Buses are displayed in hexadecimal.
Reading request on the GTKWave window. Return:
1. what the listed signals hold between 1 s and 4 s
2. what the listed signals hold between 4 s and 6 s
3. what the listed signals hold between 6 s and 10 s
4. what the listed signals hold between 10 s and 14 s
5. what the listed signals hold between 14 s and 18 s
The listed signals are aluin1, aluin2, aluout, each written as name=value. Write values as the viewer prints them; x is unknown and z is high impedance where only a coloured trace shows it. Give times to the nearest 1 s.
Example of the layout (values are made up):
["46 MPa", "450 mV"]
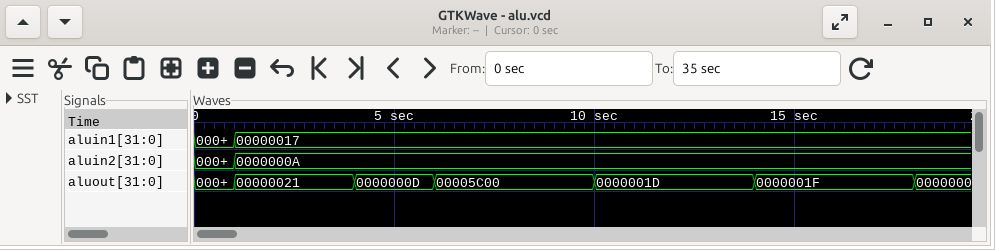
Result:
["aluin1=00000017, aluin2=0000000A, aluout=00000021", "aluin1=00000017, aluin2=0000000A, aluout=0000000D", "aluin1=00000017, aluin2=0000000A, aluout=00005C00", "aluin1=00000017, aluin2=0000000A, aluout=0000001D", "aluin1=00000017, aluin2=0000000A, aluout=0000001F"]
